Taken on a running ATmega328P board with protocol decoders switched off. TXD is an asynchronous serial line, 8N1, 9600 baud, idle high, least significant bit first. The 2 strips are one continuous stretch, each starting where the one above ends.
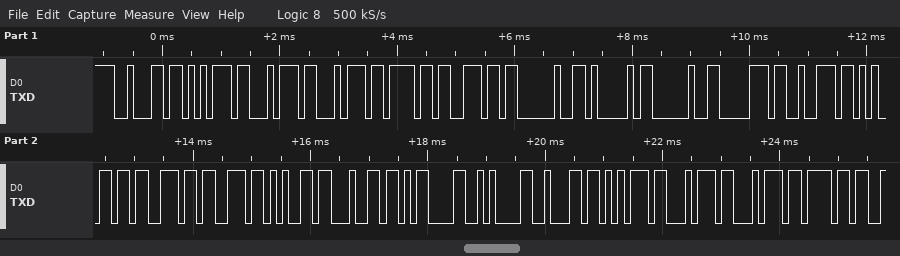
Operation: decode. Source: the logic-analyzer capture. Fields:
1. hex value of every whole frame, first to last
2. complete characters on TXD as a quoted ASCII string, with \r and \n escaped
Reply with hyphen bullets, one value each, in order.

- 62 75 74 74 6F 6E 20 41 20 70 72 65 73 73 65 64 0D 0A 62 75 74 74 6F
- "button A pressed\r\nbutto"
